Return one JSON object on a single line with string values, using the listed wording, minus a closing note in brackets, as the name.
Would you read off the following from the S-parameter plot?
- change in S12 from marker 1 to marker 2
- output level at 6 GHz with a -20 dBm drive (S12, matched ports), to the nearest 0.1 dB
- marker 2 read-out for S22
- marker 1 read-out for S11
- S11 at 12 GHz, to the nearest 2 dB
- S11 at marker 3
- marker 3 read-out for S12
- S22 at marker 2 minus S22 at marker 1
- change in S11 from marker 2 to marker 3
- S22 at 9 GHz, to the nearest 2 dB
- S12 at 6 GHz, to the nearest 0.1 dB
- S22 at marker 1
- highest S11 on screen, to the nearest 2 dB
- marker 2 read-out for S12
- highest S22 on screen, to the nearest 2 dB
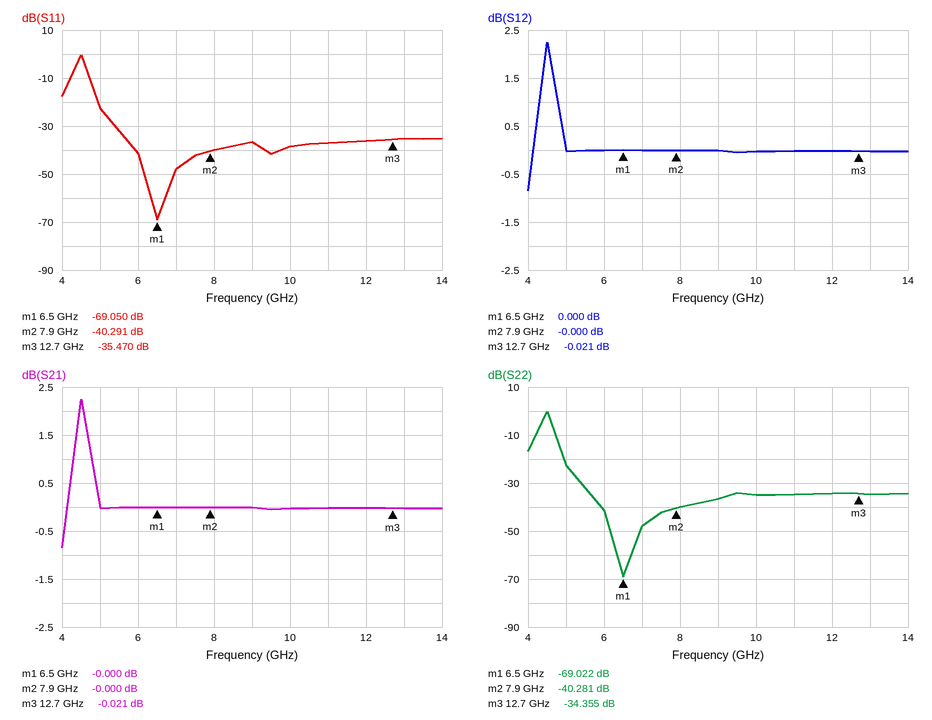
{"change in S12 from marker 1 to marker 2": "0.000 dB", "output level at 6 GHz with a -20 dBm drive (S12, matched ports), to the nearest 0.1 dB": "-20.0 dBm", "marker 2 read-out for S22": "-40.281 dB", "marker 1 read-out for S11": "-69.050 dB", "S11 at 12 GHz, to the nearest 2 dB": "-36 dB", "S11 at marker 3": "-35.470 dB", "marker 3 read-out for S12": "-0.021 dB", "S22 at marker 2 minus S22 at marker 1": "28.741 dB", "change in S11 from marker 2 to marker 3": "4.821 dB", "S22 at 9 GHz, to the nearest 2 dB": "-36 dB", "S12 at 6 GHz, to the nearest 0.1 dB": "0.0 dB", "S22 at marker 1": "-69.022 dB", "highest S11 on screen, to the nearest 2 dB": "0 dB", "marker 2 read-out for S12": "-0.000 dB", "highest S22 on screen, to the nearest 2 dB": "0 dB"}
